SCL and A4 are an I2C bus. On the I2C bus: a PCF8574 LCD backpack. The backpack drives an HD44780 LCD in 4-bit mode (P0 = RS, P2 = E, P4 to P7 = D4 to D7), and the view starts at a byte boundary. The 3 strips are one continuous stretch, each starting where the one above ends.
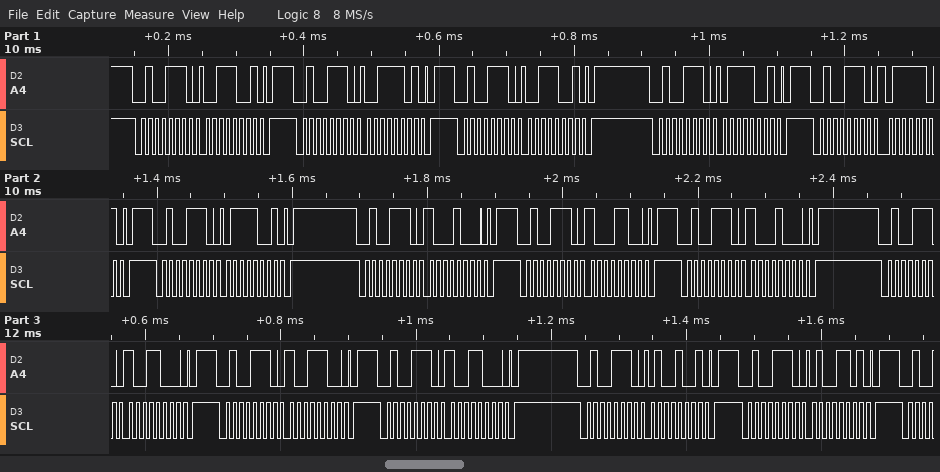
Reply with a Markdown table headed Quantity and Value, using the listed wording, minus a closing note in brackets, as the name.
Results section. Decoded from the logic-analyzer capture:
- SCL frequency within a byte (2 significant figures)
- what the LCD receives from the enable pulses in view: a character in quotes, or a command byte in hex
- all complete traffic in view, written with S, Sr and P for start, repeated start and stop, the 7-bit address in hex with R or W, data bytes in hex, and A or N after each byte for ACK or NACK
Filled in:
| Quantity | Value |
|---|---|
| SCL frequency within a byte | 100 kHz |
| what the LCD receives from the enable pulses in view: a character in quotes, or a command byte in hex | '7' 0x89 |
| all complete traffic in view, written with S, Sr and P for start, repeated start and stop, the 7-bit address in hex with R or W, data bytes in hex, and A or N after each byte for ACK or NACK | S 27W A 39 A P S 27W A 3D A P S 27W A 39 A P S 27W A 79 A P S 27W A 7D A P S 27W A 79 A P S 27W A 88 A P S 27W A 8C A P S 27W A 88 A P S 27W A 98 A P S 27W A 9C A P S 27W A 98 A P S 27W A 49 A P S 27W A 4D A P |
